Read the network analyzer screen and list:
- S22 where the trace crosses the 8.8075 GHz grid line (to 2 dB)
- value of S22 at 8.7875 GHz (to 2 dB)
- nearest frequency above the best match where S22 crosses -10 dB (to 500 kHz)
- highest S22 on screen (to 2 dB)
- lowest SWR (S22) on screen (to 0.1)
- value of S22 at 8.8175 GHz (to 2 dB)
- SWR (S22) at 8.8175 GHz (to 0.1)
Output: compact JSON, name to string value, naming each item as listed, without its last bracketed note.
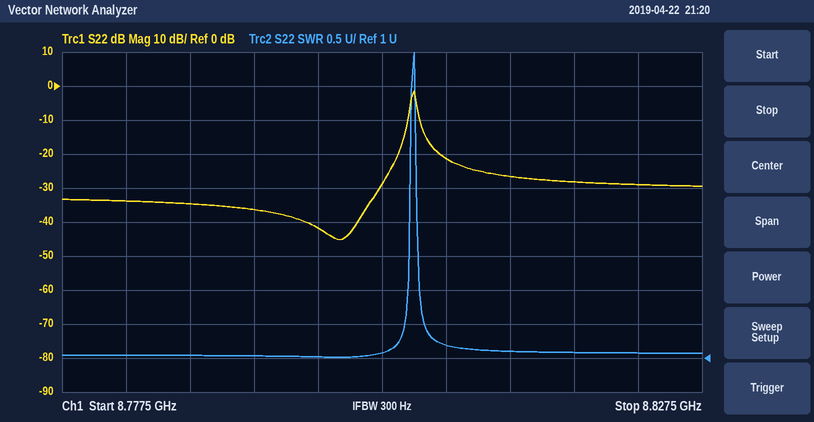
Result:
{"S22 where the trace crosses the 8.8075 GHz grid line": "-22 dB", "value of S22 at 8.7875 GHz": "-34 dB", "nearest frequency above the best match where S22 crosses -10 dB": "8.8045 GHz", "highest S22 on screen": "-2 dB", "lowest SWR (S22) on screen": "1.0", "value of S22 at 8.8175 GHz": "-28 dB", "SWR (S22) at 8.8175 GHz": "1.1"}
